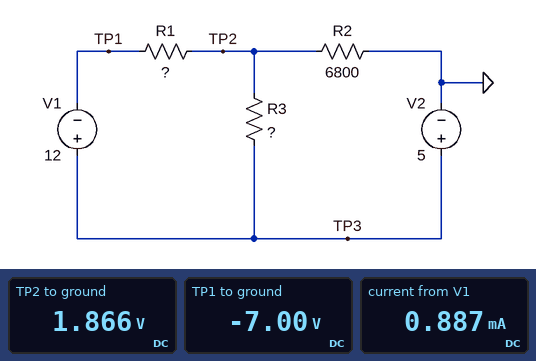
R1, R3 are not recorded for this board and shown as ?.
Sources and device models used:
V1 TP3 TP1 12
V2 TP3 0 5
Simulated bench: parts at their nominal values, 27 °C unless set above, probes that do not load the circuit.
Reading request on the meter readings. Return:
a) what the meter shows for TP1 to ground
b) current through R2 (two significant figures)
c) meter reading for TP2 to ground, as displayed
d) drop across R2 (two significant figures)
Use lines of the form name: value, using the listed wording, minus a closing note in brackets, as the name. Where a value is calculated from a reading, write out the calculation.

what the meter shows for TP1 to ground: -7.00 V
current through R2: (1.866 V) / 6.8 kΩ = 270 µA
meter reading for TP2 to ground, as displayed: 1.866 V
drop across R2: 1.866 V = 1.9 V
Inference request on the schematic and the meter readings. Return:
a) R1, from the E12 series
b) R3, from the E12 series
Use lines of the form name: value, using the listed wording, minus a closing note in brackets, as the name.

R1, from the E12 series: 10 kΩ
R3, from the E12 series: 2.7 kΩ
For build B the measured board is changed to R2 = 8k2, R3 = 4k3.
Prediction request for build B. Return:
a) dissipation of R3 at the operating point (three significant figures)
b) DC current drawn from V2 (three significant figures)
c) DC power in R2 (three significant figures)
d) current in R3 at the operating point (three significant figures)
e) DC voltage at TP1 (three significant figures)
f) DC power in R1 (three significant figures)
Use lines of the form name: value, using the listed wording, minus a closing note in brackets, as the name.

dissipation of R3 at the operating point: 3.69 mW
DC current drawn from V2: 124 µA
DC power in R2: 126 µW
current in R3 at the operating point: 926 µA
DC voltage at TP1: -7.00 V
DC power in R1: 6.43 mW
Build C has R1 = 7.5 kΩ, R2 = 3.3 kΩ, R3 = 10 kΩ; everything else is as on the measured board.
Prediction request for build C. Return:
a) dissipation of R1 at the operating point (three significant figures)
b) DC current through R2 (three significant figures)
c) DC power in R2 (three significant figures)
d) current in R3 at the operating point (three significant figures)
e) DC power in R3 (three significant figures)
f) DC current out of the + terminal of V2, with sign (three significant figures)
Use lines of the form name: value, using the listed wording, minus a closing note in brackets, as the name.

dissipation of R1 at the operating point: 5.11 mW
DC current through R2: 245 µA
DC power in R2: 198 µW
current in R3 at the operating point: 581 µA
DC power in R3: 3.37 mW
DC current out of the + terminal of V2, with sign: -245 µA
